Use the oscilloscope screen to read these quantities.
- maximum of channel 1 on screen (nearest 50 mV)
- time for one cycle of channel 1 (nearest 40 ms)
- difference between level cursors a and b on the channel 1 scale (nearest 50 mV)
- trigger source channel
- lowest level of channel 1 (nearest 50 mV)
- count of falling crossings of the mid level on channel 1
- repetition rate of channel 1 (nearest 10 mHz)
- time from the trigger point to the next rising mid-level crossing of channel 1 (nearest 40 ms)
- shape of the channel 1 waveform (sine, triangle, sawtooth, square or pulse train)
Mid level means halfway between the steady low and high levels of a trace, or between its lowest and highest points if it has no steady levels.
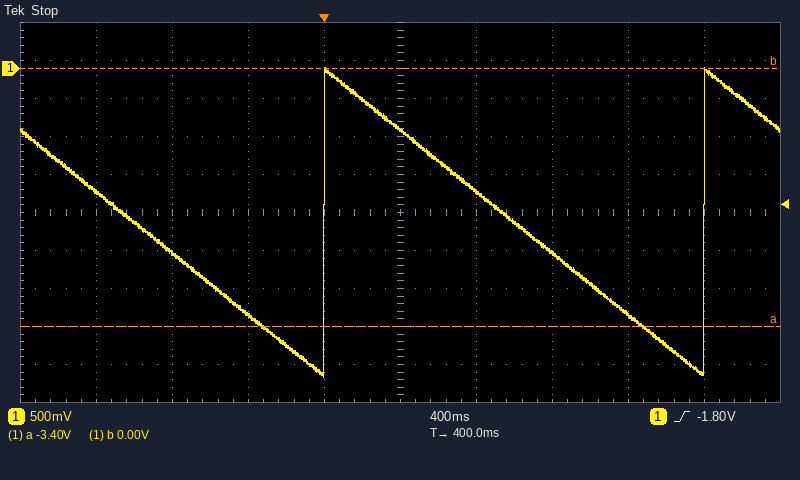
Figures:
0 mV
2.00 s
3.40 V
channel 1
-4.05 V
2
500 mHz
2.00 s
sawtooth
